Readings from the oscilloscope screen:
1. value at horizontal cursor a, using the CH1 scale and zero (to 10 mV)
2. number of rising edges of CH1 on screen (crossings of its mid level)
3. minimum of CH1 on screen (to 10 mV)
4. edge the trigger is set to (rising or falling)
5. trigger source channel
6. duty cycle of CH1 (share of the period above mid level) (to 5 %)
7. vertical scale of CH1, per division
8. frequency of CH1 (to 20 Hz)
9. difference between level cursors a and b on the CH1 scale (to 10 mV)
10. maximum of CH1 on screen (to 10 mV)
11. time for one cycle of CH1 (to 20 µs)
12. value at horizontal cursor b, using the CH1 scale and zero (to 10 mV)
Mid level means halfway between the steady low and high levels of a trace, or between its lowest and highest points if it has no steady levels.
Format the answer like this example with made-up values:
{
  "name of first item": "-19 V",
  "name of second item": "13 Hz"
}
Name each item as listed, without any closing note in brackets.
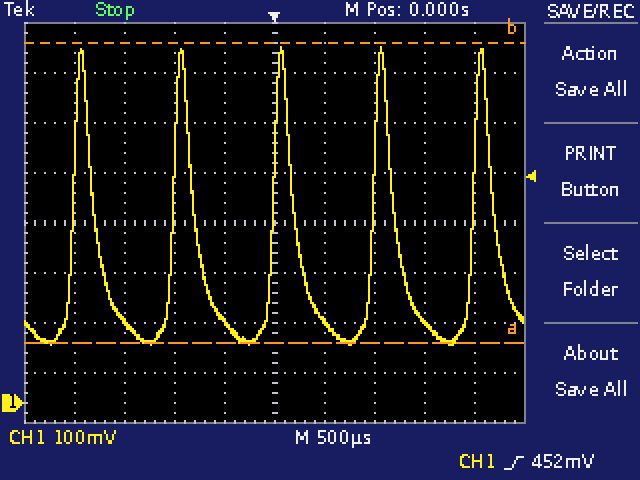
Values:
{
  "value at horizontal cursor a, using the CH1 scale and zero": "120 mV",
  "number of rising edges of CH1 on screen": "5",
  "minimum of CH1 on screen": "120 mV",
  "edge the trigger is set to": "rising",
  "trigger source channel": "CH1",
  "duty cycle of CH1 (share of the period above mid level)": "20 %",
  "vertical scale of CH1, per division": "100 mV",
  "frequency of CH1": "1.00 kHz",
  "difference between level cursors a and b on the CH1 scale": "600 mV",
  "maximum of CH1 on screen": "710 mV",
  "time for one cycle of CH1": "1.00 ms",
  "value at horizontal cursor b, using the CH1 scale and zero": "720 mV"
}
